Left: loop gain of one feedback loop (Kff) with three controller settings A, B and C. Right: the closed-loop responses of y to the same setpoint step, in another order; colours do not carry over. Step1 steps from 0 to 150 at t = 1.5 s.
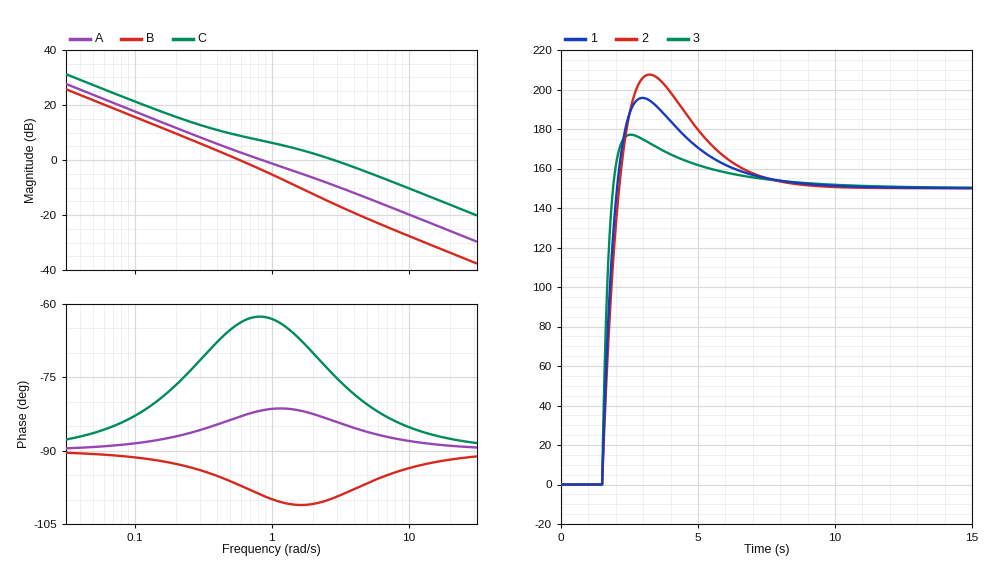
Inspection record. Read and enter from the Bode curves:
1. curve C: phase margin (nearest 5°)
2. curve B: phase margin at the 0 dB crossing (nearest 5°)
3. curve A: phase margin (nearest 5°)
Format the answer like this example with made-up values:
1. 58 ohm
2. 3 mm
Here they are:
1. 105°
2. 85°
3. 100°
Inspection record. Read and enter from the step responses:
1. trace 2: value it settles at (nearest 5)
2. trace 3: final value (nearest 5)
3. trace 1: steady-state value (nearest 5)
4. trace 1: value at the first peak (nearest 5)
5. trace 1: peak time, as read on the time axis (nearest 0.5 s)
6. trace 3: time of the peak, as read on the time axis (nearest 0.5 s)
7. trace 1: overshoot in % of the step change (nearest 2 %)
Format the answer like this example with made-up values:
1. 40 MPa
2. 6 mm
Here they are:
1. 150
2. 150
3. 150
4. 195
5. 3.0 s
6. 2.5 s
7. 30 %
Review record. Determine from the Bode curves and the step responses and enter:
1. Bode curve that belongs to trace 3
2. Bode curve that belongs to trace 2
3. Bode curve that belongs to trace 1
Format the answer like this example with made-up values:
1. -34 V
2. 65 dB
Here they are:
1. C
2. B
3. A
